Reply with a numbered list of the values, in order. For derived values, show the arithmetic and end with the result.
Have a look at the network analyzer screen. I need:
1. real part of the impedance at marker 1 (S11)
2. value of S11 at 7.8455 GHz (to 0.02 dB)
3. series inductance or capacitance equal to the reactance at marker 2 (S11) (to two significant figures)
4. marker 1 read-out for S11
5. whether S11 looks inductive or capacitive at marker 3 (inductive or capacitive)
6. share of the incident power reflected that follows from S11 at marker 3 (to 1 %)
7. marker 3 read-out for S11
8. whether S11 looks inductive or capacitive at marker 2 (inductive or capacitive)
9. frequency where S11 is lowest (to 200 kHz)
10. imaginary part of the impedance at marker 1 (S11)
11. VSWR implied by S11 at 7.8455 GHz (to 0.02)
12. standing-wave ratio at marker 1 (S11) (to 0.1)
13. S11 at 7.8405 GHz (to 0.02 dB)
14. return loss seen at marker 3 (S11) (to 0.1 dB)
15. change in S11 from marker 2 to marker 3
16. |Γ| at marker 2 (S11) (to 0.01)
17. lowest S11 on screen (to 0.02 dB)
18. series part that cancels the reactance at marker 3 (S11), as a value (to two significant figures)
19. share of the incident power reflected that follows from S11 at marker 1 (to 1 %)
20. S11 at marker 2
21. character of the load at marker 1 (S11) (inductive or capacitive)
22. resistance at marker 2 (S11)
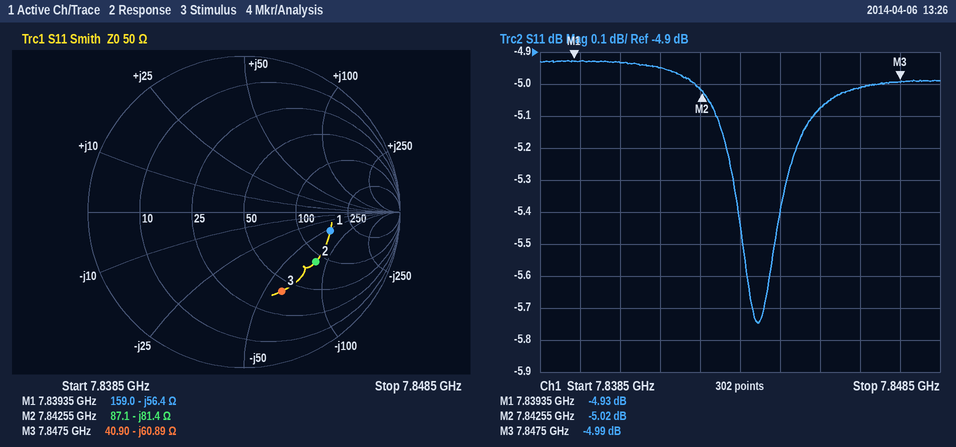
1. 159.0 Ω
2. -5.08 dB
3. C = 1/(2π × 7.84255 GHz × 81.4 Ω) ≈ 249 fF, so 250 fF to two significant figures
4. -4.93 dB
5. capacitive
6. 10^(-4.99/10) ≈ 32 %
7. -4.99 dB
8. capacitive
9. 7.8440 GHz
10. -56.4 Ω
11. |Γ| = 10^(-5.08/20) = 0.5572; VSWR = (1 + 0.5572)/(1 − 0.5572) ≈ 3.52
12. 3.6
13. -4.94 dB
14. 5.0 dB
15. -4.99 − (-5.02) = 0.03 dB
16. 0.56
17. -5.74 dB
18. L = 60.89 Ω/(2π × 7.8475 GHz) ≈ 1.2 nH
19. 10^(-4.93/10) ≈ 32 %
20. -5.02 dB
21. capacitive
22. 87.1 Ω
